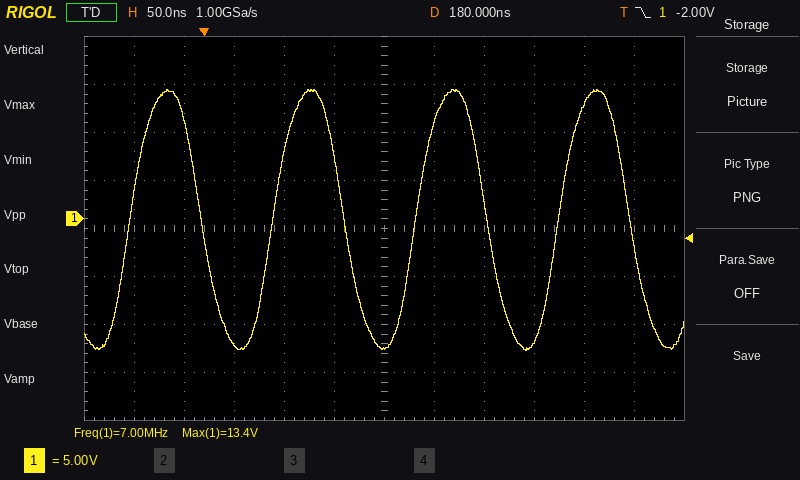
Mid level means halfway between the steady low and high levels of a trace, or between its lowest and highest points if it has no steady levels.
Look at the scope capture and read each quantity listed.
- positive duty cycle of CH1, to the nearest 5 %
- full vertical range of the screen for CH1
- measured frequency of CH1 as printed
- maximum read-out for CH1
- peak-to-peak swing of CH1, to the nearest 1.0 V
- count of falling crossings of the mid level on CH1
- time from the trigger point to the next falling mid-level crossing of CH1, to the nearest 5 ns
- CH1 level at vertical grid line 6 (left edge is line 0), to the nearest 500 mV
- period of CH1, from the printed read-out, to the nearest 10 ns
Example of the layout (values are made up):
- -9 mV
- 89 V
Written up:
- 50 %
- 40 V
- 7.00 MHz
- 13.4 V
- 27.0 V
- 4
- 140 ns
- -13.5 V
- 140 ns
